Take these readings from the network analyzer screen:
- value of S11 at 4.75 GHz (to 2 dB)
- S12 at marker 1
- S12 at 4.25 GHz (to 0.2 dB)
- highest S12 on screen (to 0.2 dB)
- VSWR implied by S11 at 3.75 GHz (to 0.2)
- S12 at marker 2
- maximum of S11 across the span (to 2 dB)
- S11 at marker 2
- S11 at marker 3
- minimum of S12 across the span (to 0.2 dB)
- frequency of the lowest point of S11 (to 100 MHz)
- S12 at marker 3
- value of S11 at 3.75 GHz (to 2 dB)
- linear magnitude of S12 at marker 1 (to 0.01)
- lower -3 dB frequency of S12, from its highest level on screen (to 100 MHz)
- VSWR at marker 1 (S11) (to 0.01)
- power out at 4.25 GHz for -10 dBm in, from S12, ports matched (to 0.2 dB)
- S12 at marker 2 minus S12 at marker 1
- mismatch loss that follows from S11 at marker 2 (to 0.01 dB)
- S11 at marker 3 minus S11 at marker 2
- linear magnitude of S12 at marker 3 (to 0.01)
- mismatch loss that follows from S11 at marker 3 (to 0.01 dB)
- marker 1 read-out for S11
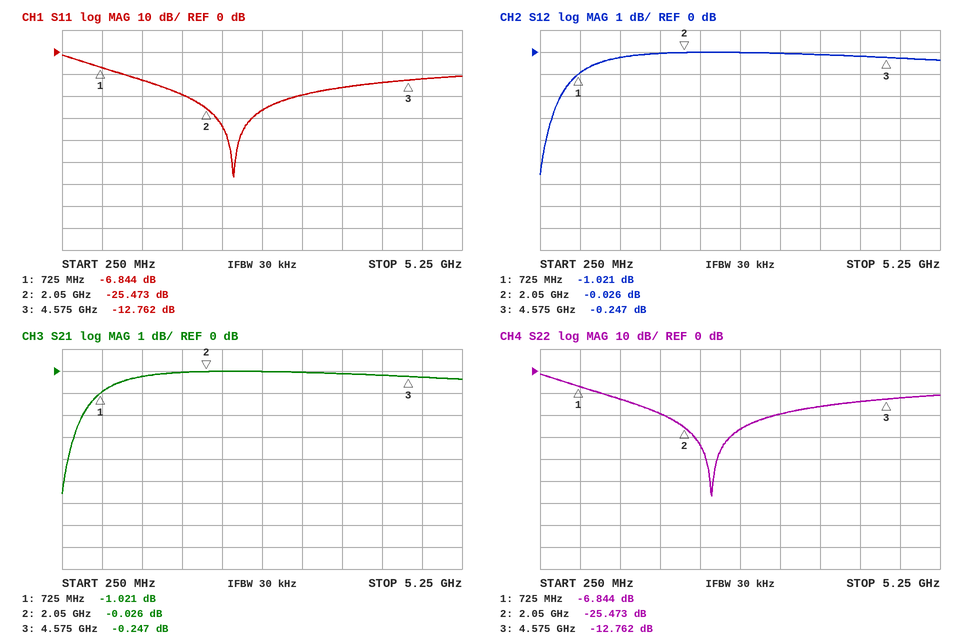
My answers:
-12 dB
-1.021 dB
-0.2 dB
0.0 dB
1.4
-0.026 dB
-2 dB
-25.473 dB
-12.762 dB
-5.6 dB
2.4 GHz
-0.247 dB
-16 dB
0.89
400 MHz
2.67
-10.2 dBm
0.995 dB
0.01 dB
12.711 dB
0.97
0.24 dB
-6.844 dB
